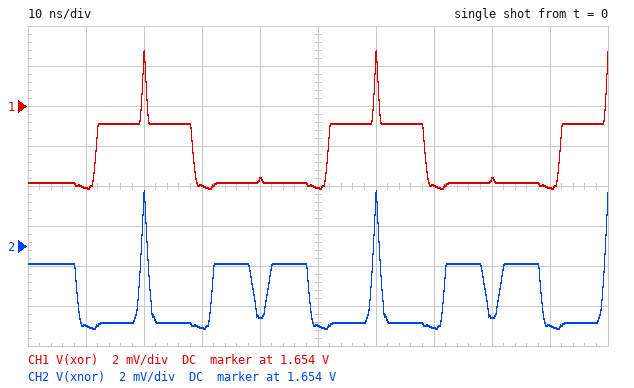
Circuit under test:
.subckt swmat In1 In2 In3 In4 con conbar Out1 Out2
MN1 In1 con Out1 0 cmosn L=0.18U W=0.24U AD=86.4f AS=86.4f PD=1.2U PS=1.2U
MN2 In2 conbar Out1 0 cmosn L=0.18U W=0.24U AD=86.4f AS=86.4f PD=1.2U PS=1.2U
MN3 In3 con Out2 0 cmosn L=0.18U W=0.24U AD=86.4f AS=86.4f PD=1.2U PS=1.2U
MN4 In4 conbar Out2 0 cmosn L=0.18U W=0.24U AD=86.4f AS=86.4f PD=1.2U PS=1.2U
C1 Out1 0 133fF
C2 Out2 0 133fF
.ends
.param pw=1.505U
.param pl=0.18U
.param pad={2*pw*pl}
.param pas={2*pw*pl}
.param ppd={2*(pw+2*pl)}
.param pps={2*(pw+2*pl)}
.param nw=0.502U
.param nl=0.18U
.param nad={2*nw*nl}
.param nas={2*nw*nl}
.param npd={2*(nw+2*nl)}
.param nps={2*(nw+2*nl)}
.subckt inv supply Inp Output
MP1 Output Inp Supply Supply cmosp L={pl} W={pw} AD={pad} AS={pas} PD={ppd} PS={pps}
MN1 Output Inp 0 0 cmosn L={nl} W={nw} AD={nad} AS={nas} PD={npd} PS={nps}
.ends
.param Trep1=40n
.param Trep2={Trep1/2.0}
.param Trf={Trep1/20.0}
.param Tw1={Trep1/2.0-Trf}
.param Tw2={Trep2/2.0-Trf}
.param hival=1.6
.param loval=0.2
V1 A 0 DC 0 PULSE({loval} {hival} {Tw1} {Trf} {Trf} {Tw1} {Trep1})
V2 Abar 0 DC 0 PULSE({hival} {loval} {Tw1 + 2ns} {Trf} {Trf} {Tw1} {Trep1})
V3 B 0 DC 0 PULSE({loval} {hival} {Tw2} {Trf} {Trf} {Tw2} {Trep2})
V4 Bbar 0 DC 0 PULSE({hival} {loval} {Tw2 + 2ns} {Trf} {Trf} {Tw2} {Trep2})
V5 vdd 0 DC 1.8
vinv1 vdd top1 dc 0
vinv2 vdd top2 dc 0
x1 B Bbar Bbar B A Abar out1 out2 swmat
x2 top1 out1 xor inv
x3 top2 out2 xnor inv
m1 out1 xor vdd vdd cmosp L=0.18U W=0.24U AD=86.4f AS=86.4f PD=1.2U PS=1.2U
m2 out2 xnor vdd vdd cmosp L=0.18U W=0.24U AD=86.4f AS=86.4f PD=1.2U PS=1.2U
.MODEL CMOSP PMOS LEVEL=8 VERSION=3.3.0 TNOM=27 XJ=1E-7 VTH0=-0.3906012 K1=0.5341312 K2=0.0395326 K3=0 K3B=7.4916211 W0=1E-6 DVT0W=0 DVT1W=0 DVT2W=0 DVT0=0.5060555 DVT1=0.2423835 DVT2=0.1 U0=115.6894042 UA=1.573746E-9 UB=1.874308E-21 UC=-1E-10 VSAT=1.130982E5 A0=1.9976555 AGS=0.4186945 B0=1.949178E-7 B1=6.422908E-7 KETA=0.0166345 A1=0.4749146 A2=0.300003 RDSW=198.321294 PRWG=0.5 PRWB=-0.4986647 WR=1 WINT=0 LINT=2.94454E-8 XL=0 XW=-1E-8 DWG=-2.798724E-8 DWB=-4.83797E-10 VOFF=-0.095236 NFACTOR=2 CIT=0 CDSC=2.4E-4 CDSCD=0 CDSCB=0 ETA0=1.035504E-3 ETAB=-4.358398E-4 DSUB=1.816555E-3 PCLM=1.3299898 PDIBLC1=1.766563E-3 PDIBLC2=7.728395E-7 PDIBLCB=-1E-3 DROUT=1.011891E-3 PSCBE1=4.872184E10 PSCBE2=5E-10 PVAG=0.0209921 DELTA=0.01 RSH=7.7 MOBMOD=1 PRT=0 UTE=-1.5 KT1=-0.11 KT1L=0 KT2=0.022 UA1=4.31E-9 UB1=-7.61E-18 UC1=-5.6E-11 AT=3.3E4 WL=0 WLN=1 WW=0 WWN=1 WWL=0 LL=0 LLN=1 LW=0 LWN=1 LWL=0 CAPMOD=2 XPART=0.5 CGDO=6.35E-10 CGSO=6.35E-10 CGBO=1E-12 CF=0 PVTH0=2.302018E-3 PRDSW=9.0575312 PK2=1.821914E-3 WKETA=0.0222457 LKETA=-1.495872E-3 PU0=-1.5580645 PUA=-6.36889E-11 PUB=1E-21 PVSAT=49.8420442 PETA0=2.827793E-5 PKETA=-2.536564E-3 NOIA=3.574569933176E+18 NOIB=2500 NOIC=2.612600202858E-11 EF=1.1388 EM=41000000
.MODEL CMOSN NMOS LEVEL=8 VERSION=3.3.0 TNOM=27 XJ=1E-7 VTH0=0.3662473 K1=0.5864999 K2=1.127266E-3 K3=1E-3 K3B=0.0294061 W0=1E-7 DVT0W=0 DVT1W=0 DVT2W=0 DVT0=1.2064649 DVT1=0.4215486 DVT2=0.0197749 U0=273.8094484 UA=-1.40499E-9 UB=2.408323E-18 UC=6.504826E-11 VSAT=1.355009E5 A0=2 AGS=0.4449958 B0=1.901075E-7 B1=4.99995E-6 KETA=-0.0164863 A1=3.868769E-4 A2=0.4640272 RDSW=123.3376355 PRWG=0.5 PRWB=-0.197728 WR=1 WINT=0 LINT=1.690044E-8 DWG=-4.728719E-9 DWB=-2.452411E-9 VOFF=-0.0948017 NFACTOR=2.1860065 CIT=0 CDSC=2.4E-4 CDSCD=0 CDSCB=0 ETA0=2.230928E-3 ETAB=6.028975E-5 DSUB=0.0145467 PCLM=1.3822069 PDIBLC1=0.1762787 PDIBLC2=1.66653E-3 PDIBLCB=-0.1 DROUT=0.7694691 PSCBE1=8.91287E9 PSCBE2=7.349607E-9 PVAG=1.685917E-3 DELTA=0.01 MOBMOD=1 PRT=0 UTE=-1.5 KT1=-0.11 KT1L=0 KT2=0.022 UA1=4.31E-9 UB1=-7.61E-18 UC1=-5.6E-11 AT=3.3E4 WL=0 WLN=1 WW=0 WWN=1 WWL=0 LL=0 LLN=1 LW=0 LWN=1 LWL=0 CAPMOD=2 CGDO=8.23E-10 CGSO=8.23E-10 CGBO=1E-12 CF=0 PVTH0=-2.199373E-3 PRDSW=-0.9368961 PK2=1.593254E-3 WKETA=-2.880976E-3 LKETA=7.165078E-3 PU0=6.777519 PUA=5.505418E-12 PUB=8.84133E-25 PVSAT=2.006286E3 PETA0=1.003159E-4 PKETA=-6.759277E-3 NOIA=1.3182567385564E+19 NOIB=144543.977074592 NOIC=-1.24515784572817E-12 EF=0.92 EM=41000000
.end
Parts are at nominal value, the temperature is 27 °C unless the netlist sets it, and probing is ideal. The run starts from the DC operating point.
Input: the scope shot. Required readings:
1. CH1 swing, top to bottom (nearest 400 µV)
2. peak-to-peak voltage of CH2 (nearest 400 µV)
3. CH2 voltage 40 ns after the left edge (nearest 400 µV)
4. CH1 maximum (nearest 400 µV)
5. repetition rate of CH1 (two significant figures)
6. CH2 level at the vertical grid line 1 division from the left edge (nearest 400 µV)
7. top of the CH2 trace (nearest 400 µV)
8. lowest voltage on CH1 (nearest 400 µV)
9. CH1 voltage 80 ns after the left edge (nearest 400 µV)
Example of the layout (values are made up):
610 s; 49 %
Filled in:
6.8 mV; 6.8 mV; 1.6504 V; 1.6568 V; 25 MHz; 1.6500 V; 1.6568 V; 1.6500 V; 1.6504 V
